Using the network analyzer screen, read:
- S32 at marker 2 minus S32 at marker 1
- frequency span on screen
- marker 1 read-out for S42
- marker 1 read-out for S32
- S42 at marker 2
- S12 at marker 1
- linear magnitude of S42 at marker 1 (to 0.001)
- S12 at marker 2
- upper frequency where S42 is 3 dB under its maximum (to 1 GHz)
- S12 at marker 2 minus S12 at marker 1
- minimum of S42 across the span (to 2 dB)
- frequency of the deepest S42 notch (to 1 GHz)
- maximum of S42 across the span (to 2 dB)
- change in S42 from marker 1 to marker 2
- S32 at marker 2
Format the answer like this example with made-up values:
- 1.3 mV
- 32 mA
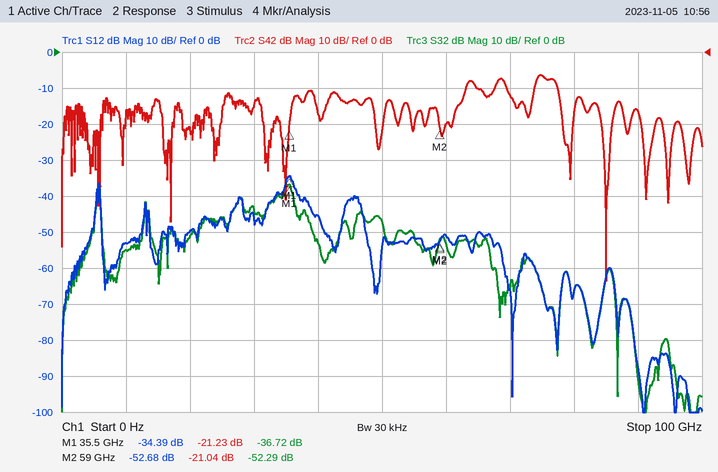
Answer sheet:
- -15.57 dB
- 100 GHz
- -21.23 dB
- -36.72 dB
- -21.04 dB
- -34.39 dB
- 0.087
- -52.68 dB
- 77 GHz
- -18.29 dB
- -64 dB
- 85 GHz
- -6 dB
- 0.19 dB
- -52.29 dB
